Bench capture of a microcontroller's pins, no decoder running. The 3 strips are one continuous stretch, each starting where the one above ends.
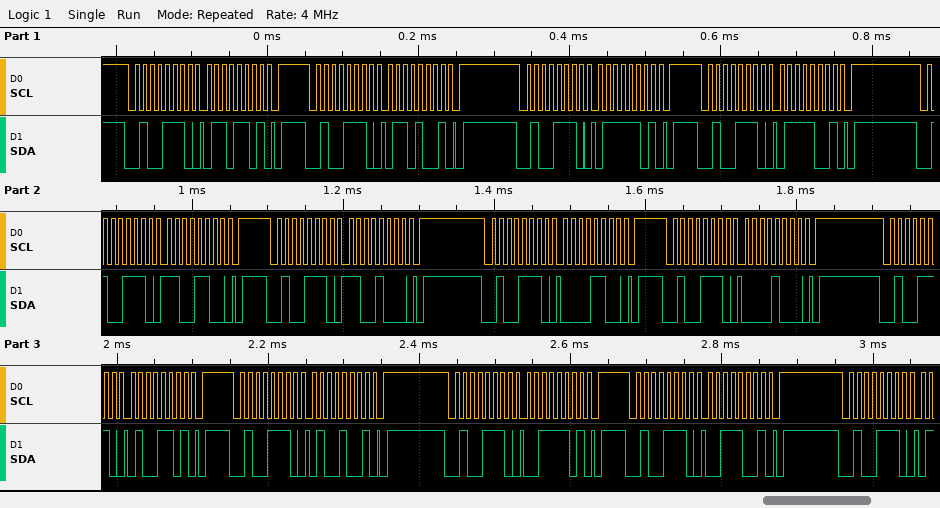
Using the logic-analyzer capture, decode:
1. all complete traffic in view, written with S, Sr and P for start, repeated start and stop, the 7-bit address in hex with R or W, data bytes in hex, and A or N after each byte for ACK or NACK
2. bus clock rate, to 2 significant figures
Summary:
S 27W A 6D A P S 27W A 69 A P S 27W A 7D A P S 27W A 79 A P S 27W A CC A P S 27W A C8 A P S 27W A 0C A P S 27W A 08 A P S 27W A 4D A P S 27W A 49 A P S 27W A 3D A P S 27W A 39 A P S 27W A
100 kHz
